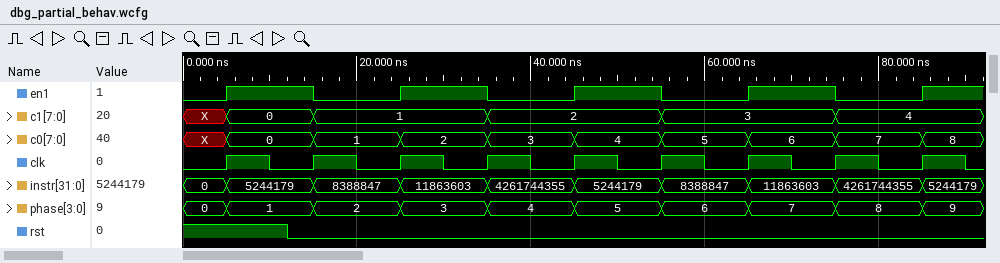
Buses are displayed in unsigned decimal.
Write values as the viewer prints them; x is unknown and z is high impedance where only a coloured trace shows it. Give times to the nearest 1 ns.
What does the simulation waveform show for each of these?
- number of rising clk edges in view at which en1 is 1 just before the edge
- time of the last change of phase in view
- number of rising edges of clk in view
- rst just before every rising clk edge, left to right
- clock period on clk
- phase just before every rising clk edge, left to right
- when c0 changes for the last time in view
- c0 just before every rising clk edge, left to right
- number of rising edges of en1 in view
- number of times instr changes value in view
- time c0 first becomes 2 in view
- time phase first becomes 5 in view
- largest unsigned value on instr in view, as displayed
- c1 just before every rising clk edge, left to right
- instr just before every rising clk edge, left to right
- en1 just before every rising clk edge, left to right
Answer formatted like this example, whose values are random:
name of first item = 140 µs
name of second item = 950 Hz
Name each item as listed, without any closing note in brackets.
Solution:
number of rising clk edges in view at which en1 is 1 just before the edge = 4
time of the last change of phase in view = 85 ns
number of rising edges of clk in view = 9
rst just before every rising clk edge, left to right = 1 0 0 0 0 0 0 0 0
clock period on clk = 10 ns
phase just before every rising clk edge, left to right = 0, 1, 2, 3, 4, 5, 6, 7, 8
when c0 changes for the last time in view = 85 ns
c0 just before every rising clk edge, left to right = X, 0, 1, 2, 3, 4, 5, 6, 7
number of rising edges of en1 in view = 5
number of times instr changes value in view = 9
time c0 first becomes 2 in view = 25 ns
time phase first becomes 5 in view = 45 ns
largest unsigned value on instr in view, as displayed = 4261744355
c1 just before every rising clk edge, left to right = X, 0, 1, 1, 2, 2, 3, 3, 4
instr just before every rising clk edge, left to right = 0, 5244179, 8388847, 11863603, 4261744355, 5244179, 8388847, 11863603, 4261744355
en1 just before every rising clk edge, left to right = 0 1 0 1 0 1 0 1 0
